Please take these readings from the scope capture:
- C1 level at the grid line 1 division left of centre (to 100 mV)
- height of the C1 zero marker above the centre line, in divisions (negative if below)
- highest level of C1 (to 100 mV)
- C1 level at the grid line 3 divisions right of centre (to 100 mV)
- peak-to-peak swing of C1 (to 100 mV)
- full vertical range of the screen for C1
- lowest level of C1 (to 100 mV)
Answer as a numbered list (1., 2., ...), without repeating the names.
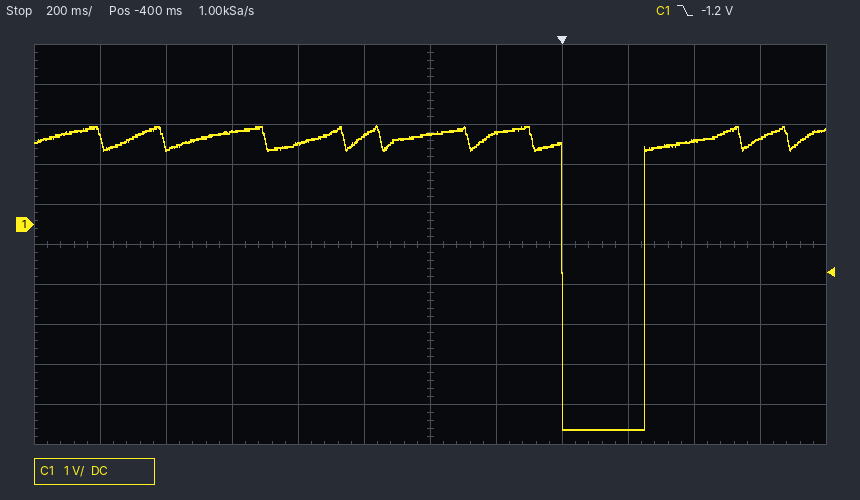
1. 2.2 V
2. +0.5 div
3. 2.5 V
4. -5.1 V
5. 7.6 V
6. 10 V
7. -5.1 V
